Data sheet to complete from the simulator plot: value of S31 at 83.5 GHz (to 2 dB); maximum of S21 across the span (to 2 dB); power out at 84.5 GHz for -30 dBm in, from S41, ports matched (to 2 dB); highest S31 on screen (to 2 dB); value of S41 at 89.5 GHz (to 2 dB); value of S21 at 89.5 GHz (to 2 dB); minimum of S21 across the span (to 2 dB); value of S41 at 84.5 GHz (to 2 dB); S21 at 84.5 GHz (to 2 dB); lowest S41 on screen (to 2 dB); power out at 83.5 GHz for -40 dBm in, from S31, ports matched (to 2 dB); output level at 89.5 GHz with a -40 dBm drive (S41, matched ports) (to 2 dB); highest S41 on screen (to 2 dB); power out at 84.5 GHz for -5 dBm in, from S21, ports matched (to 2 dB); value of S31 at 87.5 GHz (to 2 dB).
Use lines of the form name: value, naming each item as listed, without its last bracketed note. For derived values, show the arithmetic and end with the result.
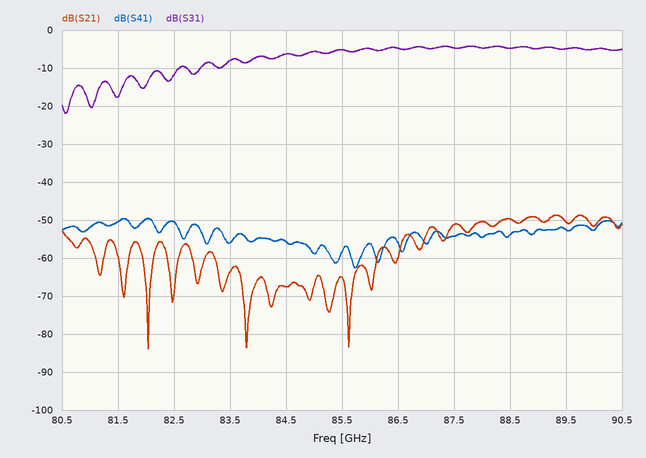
value of S31 at 83.5 GHz: -8 dB
maximum of S21 across the span: -48 dB
power out at 84.5 GHz for -30 dBm in, from S41, ports matched: -30 dBm + (-56 dB) = -86 dBm
highest S31 on screen: -4 dB
value of S41 at 89.5 GHz: -52 dB
value of S21 at 89.5 GHz: -50 dB
minimum of S21 across the span: -84 dB
value of S41 at 84.5 GHz: -56 dB
S21 at 84.5 GHz: -68 dB
lowest S41 on screen: -62 dB
power out at 83.5 GHz for -40 dBm in, from S31, ports matched: -40 dBm + (-8 dB) = -48 dBm
output level at 89.5 GHz with a -40 dBm drive (S41, matched ports): -40 dBm + (-52 dB) = -92 dBm
highest S41 on screen: -50 dB
power out at 84.5 GHz for -5 dBm in, from S21, ports matched: -5 dBm + (-68 dB) = -72 dBm
value of S31 at 87.5 GHz: -4 dB
